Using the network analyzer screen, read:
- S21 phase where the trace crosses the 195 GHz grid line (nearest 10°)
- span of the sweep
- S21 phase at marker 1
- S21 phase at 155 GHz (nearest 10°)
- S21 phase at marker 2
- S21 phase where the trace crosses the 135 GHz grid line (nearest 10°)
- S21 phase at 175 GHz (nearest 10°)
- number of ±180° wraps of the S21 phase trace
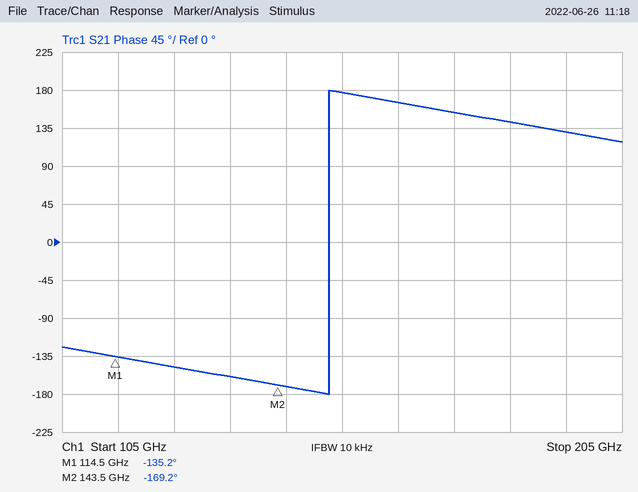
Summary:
130°
100 GHz
-135.2°
180°
-169.2°
-160°
150°
1
